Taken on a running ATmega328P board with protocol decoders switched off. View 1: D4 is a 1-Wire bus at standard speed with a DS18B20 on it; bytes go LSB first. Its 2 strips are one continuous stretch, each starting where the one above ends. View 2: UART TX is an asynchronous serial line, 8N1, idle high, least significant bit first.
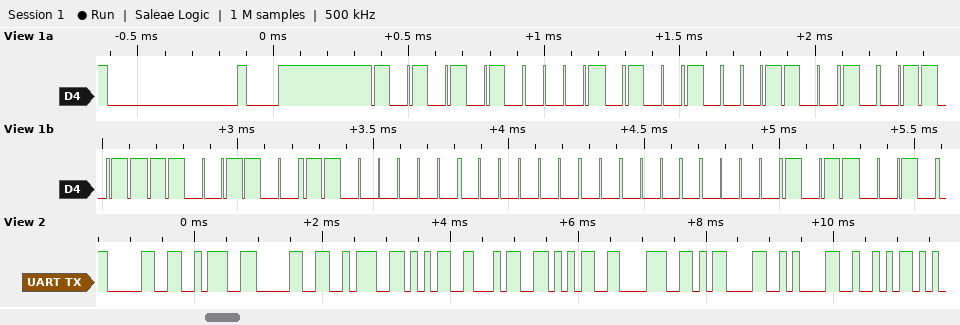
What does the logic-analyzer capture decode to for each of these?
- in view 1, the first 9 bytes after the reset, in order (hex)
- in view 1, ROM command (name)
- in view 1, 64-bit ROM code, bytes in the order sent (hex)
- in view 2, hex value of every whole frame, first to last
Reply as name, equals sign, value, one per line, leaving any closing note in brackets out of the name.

in view 1, the first 9 bytes after the reset, in order = 55 28 31 D9 33 03 00 00 4D
in view 1, ROM command = Match ROM
in view 1, 64-bit ROM code, bytes in the order sent = 28 31 D9 33 03 00 00 4D
in view 2, hex value of every whole frame, first to last = 30 3A 30 3A 35 34 35 38 0D 0A 52
